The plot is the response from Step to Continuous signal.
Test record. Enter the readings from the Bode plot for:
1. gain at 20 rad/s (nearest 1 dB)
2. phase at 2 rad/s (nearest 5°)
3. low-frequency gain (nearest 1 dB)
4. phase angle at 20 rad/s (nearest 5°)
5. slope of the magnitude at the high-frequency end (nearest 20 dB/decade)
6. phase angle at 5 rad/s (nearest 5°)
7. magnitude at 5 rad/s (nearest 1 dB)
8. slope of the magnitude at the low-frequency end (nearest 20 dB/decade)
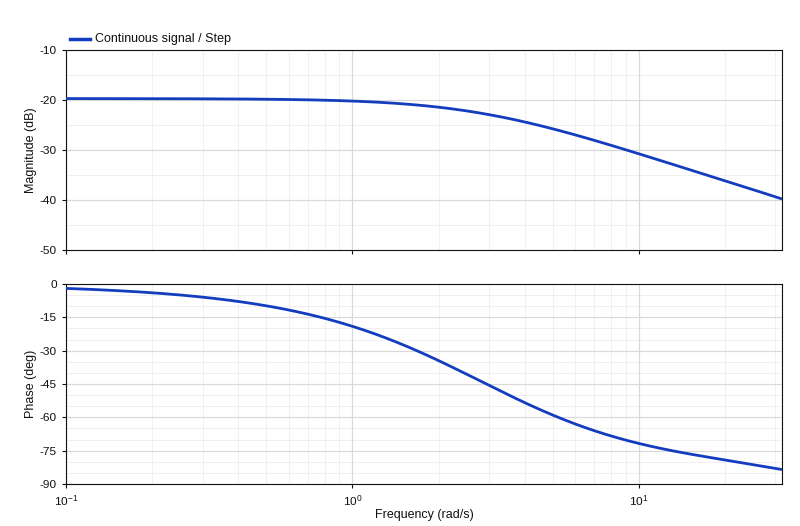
-36 dB
-35°
-20 dB
-80°
-20 dB/decade
-60°
-26 dB
0 dB/decade
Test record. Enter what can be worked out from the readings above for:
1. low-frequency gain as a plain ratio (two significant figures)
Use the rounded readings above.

0.10
